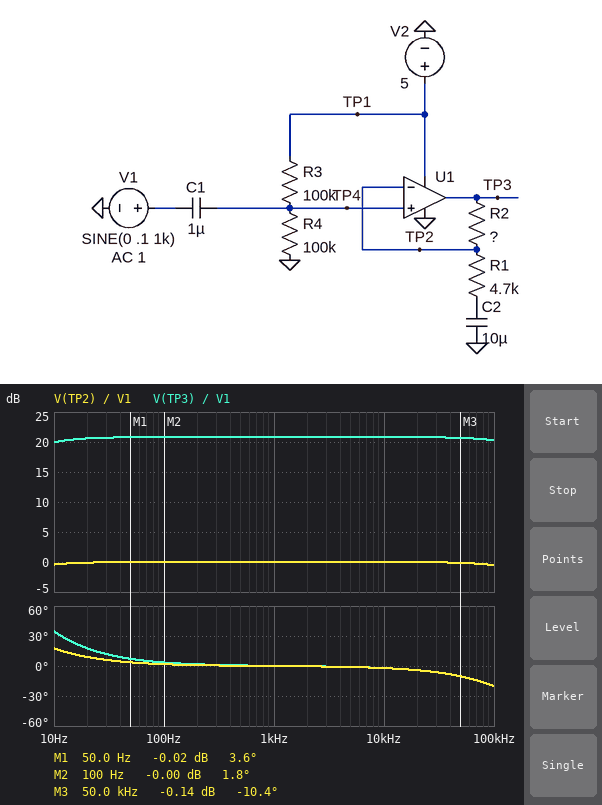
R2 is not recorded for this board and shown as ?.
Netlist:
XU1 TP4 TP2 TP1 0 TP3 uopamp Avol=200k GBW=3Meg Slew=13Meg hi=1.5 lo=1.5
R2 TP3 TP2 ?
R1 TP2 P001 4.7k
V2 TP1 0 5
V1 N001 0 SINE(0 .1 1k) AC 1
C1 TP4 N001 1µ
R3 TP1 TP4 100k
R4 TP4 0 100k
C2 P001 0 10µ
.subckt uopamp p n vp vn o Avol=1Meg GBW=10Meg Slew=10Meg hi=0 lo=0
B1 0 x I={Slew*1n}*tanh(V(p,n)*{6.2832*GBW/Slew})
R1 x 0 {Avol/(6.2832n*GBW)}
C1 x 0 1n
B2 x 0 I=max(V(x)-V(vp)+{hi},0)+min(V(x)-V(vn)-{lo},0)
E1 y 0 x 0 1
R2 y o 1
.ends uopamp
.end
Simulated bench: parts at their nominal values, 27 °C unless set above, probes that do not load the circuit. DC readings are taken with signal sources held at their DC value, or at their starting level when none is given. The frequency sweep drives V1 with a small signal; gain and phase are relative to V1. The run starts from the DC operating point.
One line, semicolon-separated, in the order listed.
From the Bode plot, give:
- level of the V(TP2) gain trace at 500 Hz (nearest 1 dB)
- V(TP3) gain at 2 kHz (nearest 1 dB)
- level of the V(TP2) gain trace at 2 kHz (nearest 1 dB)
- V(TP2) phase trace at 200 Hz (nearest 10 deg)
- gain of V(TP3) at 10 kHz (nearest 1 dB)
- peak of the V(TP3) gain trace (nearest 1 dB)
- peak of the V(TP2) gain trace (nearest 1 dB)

0 dB; 21 dB; 0 dB; 0 deg; 21 dB; 21 dB; 0 dB
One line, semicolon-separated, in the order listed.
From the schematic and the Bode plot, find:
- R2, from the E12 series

47 kΩ
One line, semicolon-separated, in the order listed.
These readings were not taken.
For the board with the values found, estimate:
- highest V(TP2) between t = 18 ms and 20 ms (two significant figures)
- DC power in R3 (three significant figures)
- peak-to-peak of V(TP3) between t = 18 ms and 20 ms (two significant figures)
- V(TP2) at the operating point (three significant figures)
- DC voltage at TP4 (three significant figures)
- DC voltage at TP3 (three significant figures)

2.6 V; 62.5 µW; 2.0 V; 2.50 V; 2.50 V; 2.50 V
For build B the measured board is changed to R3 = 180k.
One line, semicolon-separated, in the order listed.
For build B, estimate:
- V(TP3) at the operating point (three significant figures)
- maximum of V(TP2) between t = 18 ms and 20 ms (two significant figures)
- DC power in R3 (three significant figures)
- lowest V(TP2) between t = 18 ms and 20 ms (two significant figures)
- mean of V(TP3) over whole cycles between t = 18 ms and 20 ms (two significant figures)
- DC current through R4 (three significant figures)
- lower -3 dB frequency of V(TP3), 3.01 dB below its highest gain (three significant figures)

1.79 V; 1.9 V; 57.4 µW; 1.8 V; 2.0 V; 17.9 µA; 4.56 Hz
